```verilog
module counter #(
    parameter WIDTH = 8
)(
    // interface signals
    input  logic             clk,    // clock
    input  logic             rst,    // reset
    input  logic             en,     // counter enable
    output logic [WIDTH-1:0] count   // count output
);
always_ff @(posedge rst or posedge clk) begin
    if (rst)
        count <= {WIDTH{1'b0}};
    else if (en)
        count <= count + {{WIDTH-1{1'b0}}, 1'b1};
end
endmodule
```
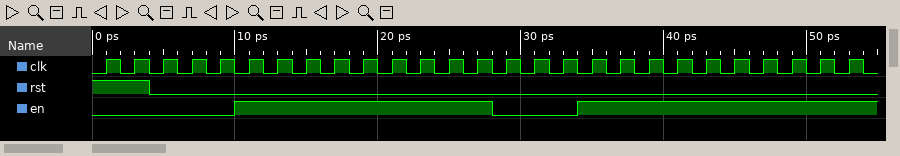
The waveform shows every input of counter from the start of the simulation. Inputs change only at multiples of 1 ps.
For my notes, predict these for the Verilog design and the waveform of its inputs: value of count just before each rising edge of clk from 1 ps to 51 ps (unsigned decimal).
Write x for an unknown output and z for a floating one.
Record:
0, 0, 0, 0, 0, 0, 1, 2, 3, 4, 5, 6, 7, 8, 9, 9, 9, 9, 10, 11, 12, 13, 14, 15, 16, 17
